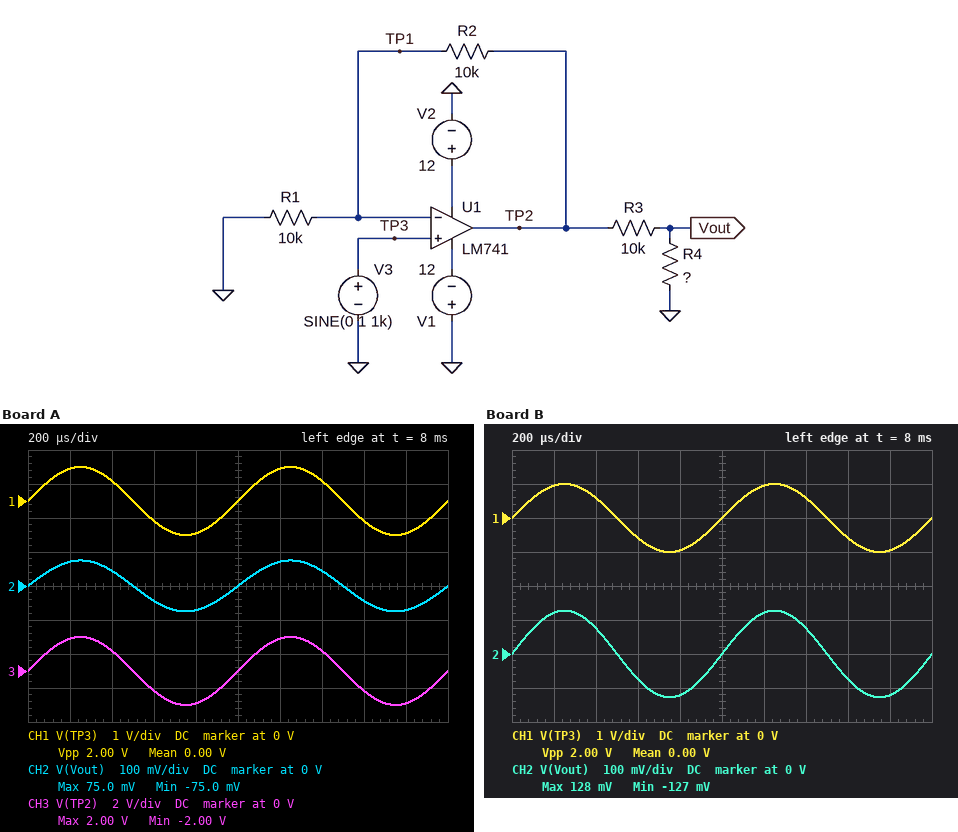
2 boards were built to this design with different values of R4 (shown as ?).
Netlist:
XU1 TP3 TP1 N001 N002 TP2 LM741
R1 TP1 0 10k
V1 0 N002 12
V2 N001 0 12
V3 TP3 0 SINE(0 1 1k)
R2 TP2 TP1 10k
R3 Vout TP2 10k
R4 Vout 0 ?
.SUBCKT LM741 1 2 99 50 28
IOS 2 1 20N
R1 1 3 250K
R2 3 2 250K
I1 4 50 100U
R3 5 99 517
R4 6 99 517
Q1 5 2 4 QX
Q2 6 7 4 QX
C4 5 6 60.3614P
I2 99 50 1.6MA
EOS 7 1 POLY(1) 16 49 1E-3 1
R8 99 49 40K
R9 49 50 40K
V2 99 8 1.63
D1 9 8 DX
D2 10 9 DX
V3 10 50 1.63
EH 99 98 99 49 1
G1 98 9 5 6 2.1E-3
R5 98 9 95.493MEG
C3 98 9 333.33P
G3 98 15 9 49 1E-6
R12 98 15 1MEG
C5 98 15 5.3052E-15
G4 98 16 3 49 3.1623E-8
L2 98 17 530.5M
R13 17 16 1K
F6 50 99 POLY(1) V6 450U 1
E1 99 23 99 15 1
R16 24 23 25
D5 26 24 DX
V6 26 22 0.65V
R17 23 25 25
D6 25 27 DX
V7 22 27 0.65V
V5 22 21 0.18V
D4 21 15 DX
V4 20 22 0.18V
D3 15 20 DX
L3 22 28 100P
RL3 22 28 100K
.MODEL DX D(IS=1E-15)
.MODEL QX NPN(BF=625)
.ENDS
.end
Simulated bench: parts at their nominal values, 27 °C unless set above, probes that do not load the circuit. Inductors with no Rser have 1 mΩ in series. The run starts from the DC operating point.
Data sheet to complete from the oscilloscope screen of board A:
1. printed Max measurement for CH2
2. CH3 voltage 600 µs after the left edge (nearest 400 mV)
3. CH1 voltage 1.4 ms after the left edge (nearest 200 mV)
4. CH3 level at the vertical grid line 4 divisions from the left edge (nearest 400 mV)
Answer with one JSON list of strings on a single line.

["75.0 mV", "-1.2 V", "600 mV", "-2.0 V"]
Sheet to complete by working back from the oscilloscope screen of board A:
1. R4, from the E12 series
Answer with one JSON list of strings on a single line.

["390 Ω"]
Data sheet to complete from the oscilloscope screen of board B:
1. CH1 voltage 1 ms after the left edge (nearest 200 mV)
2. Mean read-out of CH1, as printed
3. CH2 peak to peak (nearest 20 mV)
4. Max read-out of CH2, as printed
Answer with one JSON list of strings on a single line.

["0 V", "0.00 V", "260 mV", "128 mV"]
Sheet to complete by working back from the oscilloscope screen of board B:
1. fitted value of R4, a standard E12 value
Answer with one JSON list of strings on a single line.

["680 Ω"]
